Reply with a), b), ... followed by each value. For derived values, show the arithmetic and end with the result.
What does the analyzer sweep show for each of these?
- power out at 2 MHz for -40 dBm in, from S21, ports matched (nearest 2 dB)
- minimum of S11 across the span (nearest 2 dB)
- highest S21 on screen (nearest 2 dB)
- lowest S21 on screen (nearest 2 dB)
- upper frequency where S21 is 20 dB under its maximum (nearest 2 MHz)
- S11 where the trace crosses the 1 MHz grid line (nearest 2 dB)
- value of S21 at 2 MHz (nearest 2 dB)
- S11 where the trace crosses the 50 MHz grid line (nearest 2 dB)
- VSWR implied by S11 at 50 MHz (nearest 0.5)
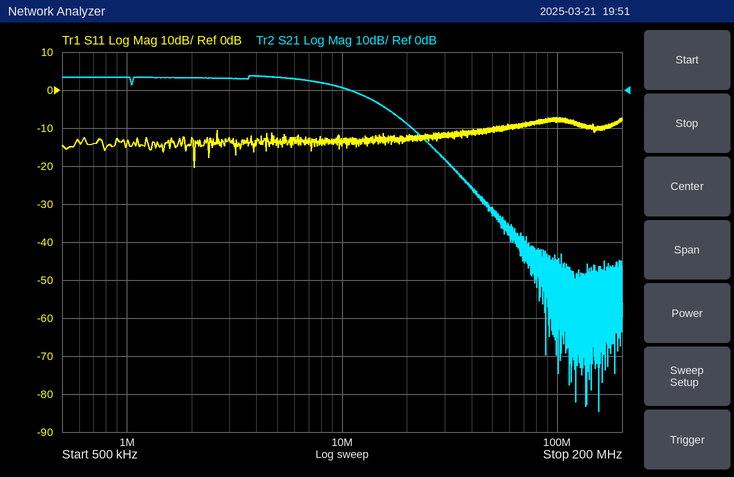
a) -40 dBm + (4 dB) = -36 dBm
b) -20 dB
c) 4 dB
d) -84 dB
e) 28 MHz
f) -14 dB
g) 4 dB
h) -10 dB
i) |Γ| = 10^(-10/20) = 0.3162; VSWR = (1 + 0.3162)/(1 − 0.3162) ≈ 1.92, so 2.0 to the nearest 0.5
